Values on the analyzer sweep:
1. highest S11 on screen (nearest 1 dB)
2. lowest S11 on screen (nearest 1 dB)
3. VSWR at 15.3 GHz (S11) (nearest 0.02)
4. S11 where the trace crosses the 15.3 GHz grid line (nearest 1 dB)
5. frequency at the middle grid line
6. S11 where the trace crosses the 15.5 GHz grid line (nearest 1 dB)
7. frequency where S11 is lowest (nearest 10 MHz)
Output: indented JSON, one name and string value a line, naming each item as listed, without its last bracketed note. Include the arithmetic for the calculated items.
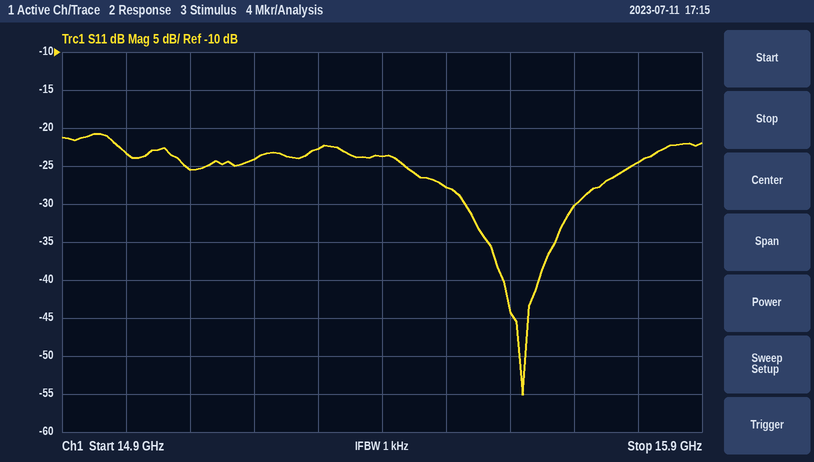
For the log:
{
  "highest S11 on screen": "-21 dB",
  "lowest S11 on screen": "-55 dB",
  "VSWR at 15.3 GHz (S11)": "|Γ| = 10^(-23/20) = 0.0708; VSWR = (1 + 0.0708)/(1 − 0.0708) ≈ 1.15, so 1.16 to the nearest 0.02",
  "S11 where the trace crosses the 15.3 GHz grid line": "-23 dB",
  "frequency at the middle grid line": "15.4 GHz",
  "S11 where the trace crosses the 15.5 GHz grid line": "-28 dB",
  "frequency where S11 is lowest": "15.62 GHz"
}
